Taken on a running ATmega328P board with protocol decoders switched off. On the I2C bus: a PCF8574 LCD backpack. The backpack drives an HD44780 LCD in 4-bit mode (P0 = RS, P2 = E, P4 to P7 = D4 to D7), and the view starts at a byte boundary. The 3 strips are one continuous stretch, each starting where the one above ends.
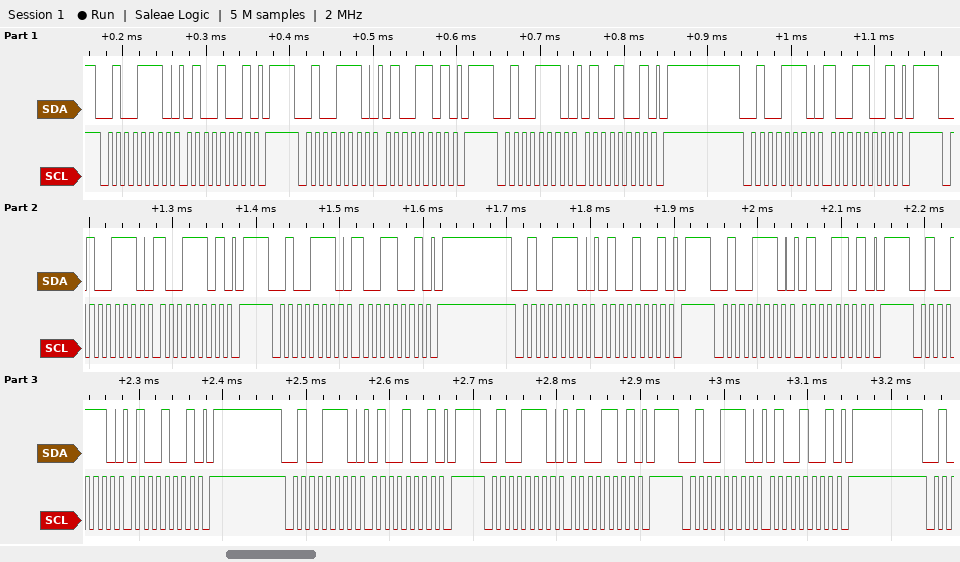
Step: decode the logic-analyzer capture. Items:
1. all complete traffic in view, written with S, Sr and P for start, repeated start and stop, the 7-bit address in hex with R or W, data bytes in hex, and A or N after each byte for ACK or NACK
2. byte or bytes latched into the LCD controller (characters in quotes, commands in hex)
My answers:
S 27W A 49 A P S 27W A 4D A P S 27W A 49 A P S 27W A 99 A P S 27W A 9D A P S 27W A 99 A P S 27W A 49 A P S 27W A 4D A P S 27W A 49 A P S 27W A 49 A P S 27W A 4D A P S 27W A 49 A P
'I' 'D'
